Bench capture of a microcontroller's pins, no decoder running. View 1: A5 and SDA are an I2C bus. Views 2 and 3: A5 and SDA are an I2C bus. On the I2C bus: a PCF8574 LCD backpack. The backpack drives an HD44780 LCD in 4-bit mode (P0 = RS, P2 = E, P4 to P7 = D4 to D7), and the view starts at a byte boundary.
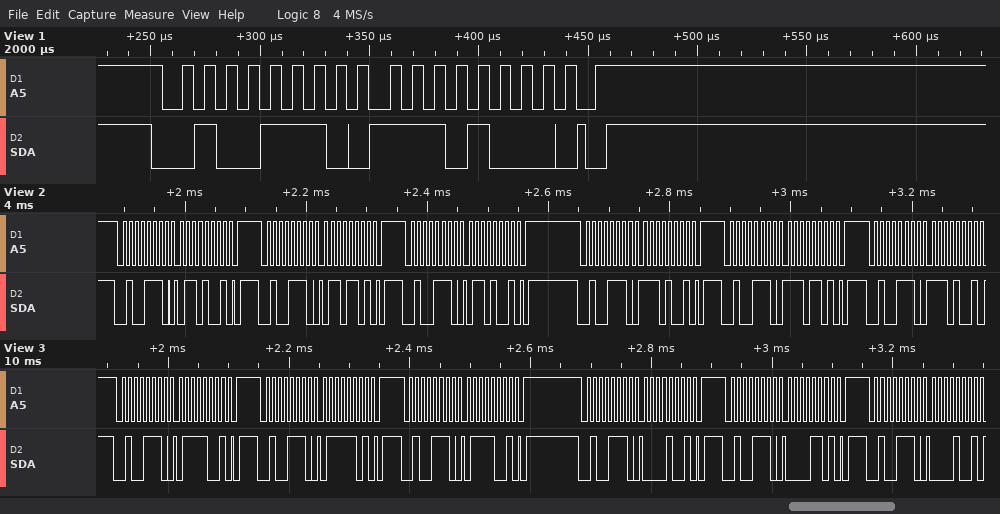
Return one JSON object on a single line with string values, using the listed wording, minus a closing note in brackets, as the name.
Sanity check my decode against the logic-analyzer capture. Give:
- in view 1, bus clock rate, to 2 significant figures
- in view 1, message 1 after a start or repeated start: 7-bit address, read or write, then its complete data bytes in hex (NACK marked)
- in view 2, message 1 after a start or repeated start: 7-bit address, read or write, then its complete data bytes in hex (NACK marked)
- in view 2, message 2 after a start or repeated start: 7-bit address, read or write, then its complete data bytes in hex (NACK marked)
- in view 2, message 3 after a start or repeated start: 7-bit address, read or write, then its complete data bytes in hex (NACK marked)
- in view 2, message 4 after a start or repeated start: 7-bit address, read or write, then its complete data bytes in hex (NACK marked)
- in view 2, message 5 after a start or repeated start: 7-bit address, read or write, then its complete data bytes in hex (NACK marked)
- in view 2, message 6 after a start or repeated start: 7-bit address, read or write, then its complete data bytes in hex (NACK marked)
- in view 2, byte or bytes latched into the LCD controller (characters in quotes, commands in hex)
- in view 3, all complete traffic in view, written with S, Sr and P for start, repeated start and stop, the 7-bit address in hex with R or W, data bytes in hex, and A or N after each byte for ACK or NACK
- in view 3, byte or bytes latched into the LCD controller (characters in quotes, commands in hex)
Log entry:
{"in view 1, bus clock rate, to 2 significant figures": "100 kHz", "in view 1, message 1 after a start or repeated start: 7-bit address, read or write, then its complete data bytes in hex": "0x27 write: E8", "in view 2, message 1 after a start or repeated start: 7-bit address, read or write, then its complete data bytes in hex": "0x27 write: 69", "in view 2, message 2 after a start or repeated start: 7-bit address, read or write, then its complete data bytes in hex": "0x27 write: 6D", "in view 2, message 3 after a start or repeated start: 7-bit address, read or write, then its complete data bytes in hex": "0x27 write: 69", "in view 2, message 4 after a start or repeated start: 7-bit address, read or write, then its complete data bytes in hex": "0x27 write: E9", "in view 2, message 5 after a start or repeated start: 7-bit address, read or write, then its complete data bytes in hex": "0x27 write: ED", "in view 2, message 6 after a start or repeated start: 7-bit address, read or write, then its complete data bytes in hex": "0x27 write: E9", "in view 2, byte or bytes latched into the LCD controller": "'n'", "in view 3, all complete traffic in view, written with S, Sr and P for start, repeated start and stop, the 7-bit address in hex with R or W, data bytes in hex, and A or N after each byte for ACK or NACK": "S 27W A 79 A P S 27W A 7D A P S 27W A 79 A P S 27W A 09 A P S 27W A 0D A P S 27W A 09 A", "in view 3, byte or bytes latched into the LCD controller": "'p'"}
